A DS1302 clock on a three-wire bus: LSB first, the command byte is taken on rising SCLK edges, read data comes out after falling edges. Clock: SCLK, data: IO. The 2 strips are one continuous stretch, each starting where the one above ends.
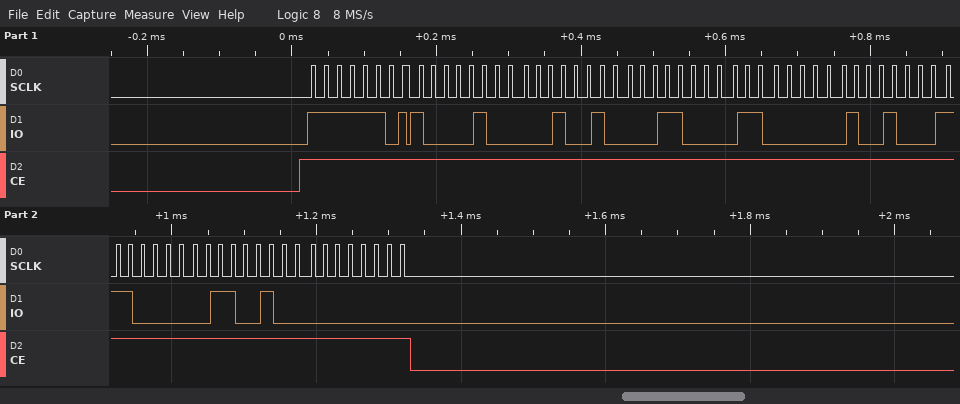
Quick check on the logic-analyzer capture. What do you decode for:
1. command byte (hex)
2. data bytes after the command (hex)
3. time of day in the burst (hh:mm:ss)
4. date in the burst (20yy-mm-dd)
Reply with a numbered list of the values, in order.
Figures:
1. 0xBF
2. 21 48 18 06 12 07 26 00
3. 18:48:21
4. 2026-12-06
